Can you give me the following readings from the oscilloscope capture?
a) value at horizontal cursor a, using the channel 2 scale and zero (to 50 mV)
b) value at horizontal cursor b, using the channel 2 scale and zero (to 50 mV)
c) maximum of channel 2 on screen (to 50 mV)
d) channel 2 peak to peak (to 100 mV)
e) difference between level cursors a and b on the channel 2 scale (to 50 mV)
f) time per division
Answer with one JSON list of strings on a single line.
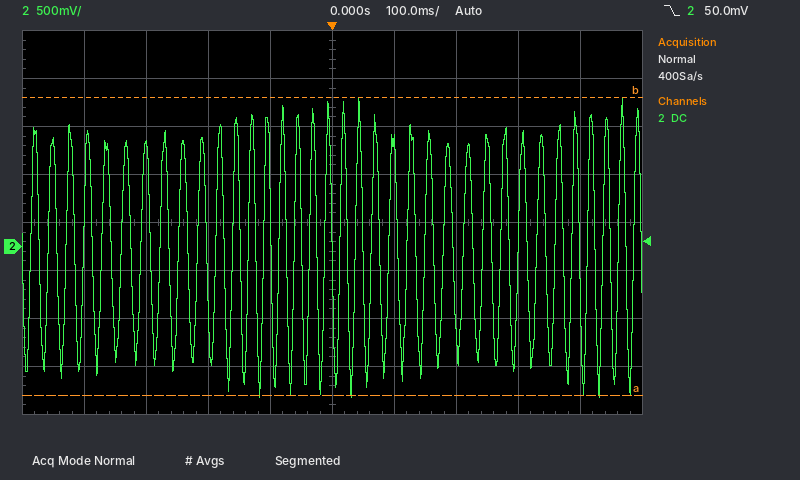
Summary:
["-1.55 V", "1.55 V", "1.55 V", "3.10 V", "3.10 V", "100 ms"]
